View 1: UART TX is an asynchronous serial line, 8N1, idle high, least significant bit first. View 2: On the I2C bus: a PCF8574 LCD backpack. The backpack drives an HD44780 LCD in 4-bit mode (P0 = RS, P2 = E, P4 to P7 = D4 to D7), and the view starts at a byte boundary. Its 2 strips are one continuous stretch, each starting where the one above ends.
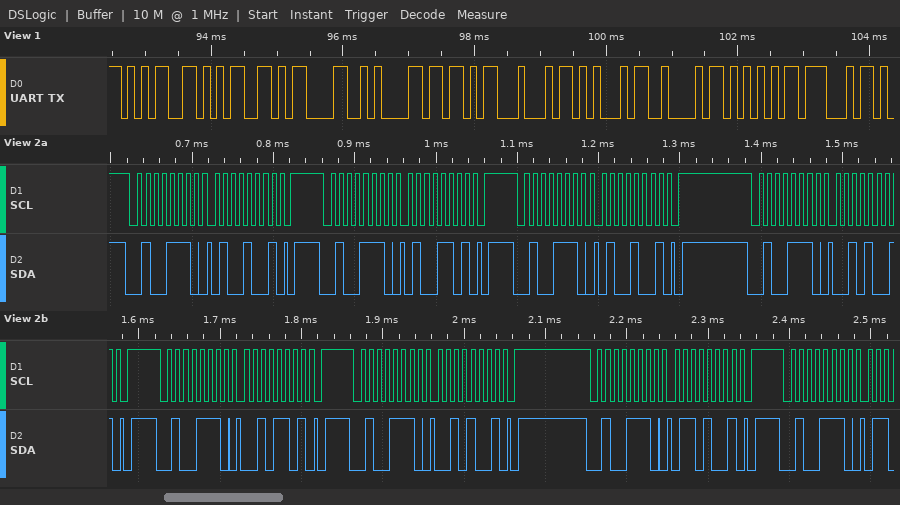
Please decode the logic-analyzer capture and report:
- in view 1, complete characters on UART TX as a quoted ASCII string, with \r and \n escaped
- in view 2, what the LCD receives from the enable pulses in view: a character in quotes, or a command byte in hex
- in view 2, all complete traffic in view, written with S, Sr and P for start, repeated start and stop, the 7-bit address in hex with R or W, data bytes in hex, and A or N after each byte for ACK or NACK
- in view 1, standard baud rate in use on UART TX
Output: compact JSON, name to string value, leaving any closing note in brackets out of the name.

{"in view 1, complete characters on UART TX as a quoted ASCII string, with \\r and \\n escaped": "\"55\\r\\n[DEBUG\"", "in view 2, what the LCD receives from the enable pulses in view: a character in quotes, or a command byte in hex": "'B'", "in view 2, all complete traffic in view, written with S, Sr and P for start, repeated start and stop, the 7-bit address in hex with R or W, data bytes in hex, and A or N after each byte for ACK or NACK": "S 27W A 49 A P S 27W A 4D A P S 27W A 49 A P S 27W A 29 A P S 27W A 2D A P S 27W A 29 A P S 27W A 69 A P S 27W A", "in view 1, standard baud rate in use on UART TX": "9600 baud"}
